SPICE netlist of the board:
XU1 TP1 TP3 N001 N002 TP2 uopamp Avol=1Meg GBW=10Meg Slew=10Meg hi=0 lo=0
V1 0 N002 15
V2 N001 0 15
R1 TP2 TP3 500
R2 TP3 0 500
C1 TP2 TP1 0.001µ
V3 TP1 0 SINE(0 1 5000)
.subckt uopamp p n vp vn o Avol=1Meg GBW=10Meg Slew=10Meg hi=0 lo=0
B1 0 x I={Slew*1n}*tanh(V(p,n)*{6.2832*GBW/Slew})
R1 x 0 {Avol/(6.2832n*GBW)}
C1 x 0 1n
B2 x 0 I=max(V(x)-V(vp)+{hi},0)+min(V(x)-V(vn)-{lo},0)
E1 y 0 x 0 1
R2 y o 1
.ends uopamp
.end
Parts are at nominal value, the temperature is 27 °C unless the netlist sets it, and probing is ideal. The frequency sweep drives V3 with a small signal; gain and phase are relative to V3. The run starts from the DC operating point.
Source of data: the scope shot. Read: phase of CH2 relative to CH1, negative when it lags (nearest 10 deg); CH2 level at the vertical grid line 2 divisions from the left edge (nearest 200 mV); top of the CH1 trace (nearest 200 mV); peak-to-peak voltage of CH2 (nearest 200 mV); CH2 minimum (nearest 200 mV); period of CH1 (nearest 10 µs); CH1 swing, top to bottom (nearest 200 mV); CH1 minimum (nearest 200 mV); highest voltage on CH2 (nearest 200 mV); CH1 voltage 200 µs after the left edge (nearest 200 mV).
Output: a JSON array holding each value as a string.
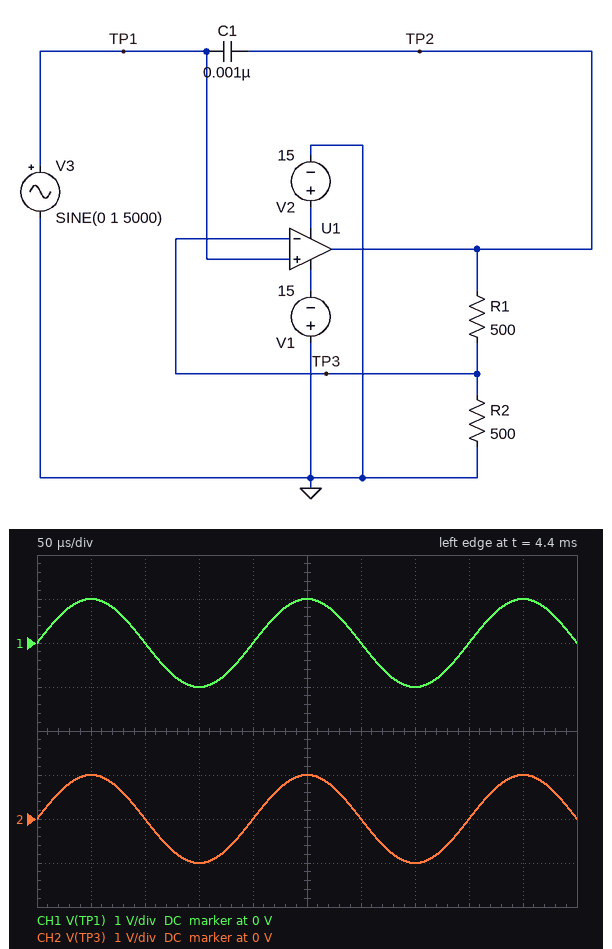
["0 deg", "0 V", "1.0 V", "2.0 V", "-1.0 V", "200 µs", "2.0 V", "-1.0 V", "1.0 V", "0 V"]
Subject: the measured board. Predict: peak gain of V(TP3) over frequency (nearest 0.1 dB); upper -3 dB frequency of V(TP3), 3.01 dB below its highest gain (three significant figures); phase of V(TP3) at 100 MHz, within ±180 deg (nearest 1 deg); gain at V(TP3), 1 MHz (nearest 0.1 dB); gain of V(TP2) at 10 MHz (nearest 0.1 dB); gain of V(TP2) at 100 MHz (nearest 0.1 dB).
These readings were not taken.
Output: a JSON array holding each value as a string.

["0 dB", "4.99 MHz", "60 deg", "-0.2 dB", "-1.3 dB", "-6.8 dB"]
